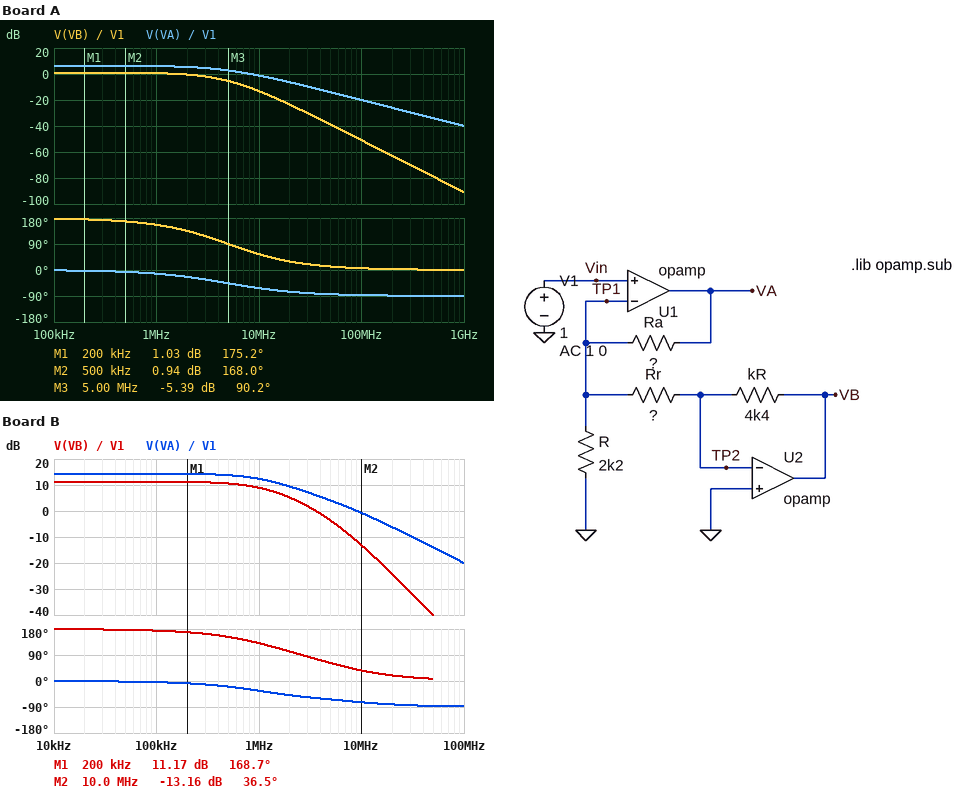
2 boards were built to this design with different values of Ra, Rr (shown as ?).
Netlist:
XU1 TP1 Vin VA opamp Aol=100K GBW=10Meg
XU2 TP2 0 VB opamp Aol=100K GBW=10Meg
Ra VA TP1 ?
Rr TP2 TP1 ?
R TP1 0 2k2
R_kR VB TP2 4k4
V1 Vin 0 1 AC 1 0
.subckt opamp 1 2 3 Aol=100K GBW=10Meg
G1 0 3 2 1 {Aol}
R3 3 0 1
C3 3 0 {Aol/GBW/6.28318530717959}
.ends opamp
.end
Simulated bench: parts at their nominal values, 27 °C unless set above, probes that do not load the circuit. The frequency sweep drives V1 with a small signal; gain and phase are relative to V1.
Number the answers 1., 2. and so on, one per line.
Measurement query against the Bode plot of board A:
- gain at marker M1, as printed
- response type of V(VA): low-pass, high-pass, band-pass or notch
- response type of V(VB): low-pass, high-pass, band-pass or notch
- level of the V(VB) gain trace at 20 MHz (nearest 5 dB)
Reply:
1. 1.03 dB
2. low-pass
3. low-pass
4. -25 dB
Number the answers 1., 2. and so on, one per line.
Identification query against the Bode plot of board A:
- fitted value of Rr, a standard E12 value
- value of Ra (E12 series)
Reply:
1. 3.9 kΩ
2. 1.5 kΩ
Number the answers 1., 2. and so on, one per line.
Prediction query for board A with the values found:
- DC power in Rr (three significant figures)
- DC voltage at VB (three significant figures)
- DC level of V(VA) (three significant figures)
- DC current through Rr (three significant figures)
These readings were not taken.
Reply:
1. 256 µW
2. -1.13 V
3. 2.07 V
4. 256 µA
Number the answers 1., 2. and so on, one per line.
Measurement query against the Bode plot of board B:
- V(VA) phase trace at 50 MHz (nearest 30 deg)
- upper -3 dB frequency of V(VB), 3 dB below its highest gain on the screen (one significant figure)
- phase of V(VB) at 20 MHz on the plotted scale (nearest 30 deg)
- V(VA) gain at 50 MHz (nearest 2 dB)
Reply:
1. -90 deg
2. 1 MHz
3. 30 deg
4. -14 dB
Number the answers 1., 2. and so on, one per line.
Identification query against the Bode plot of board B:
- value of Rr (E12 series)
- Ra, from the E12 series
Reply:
1. 1.2 kΩ
2. 3.3 kΩ
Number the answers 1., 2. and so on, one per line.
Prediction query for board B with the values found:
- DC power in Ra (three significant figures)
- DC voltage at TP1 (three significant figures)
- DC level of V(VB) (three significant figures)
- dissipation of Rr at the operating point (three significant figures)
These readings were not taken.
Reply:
1. 5.47 mW
2. 1.00 V
3. -3.67 V
4. 833 µW
